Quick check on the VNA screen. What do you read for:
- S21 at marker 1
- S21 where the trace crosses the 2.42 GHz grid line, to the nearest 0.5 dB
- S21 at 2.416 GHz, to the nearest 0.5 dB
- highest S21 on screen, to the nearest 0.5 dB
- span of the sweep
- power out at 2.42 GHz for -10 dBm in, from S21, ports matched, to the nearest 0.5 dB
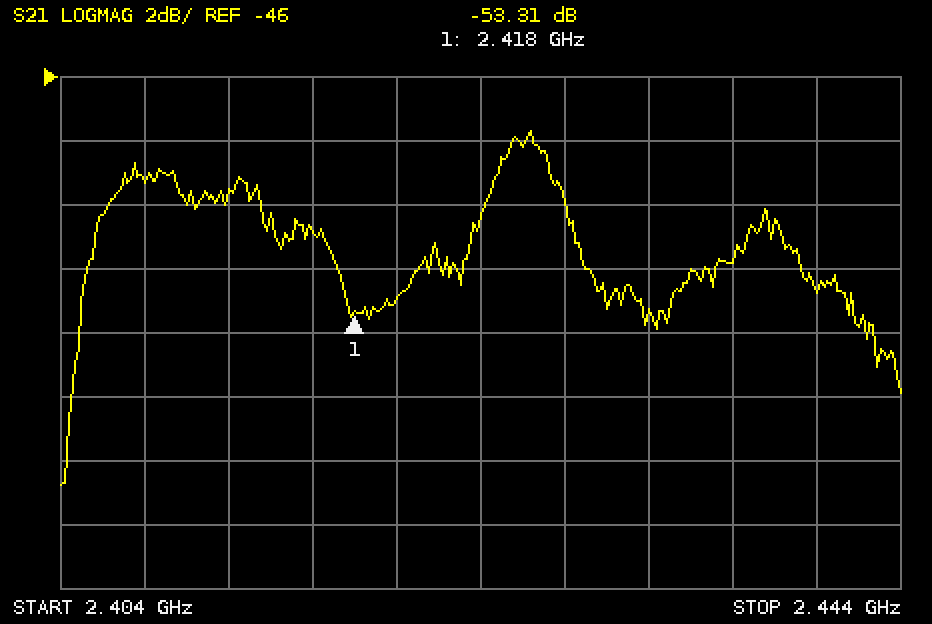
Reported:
-53.31 dB
-53.0 dB
-51.0 dB
-47.5 dB
40 MHz
-63.0 dBm
